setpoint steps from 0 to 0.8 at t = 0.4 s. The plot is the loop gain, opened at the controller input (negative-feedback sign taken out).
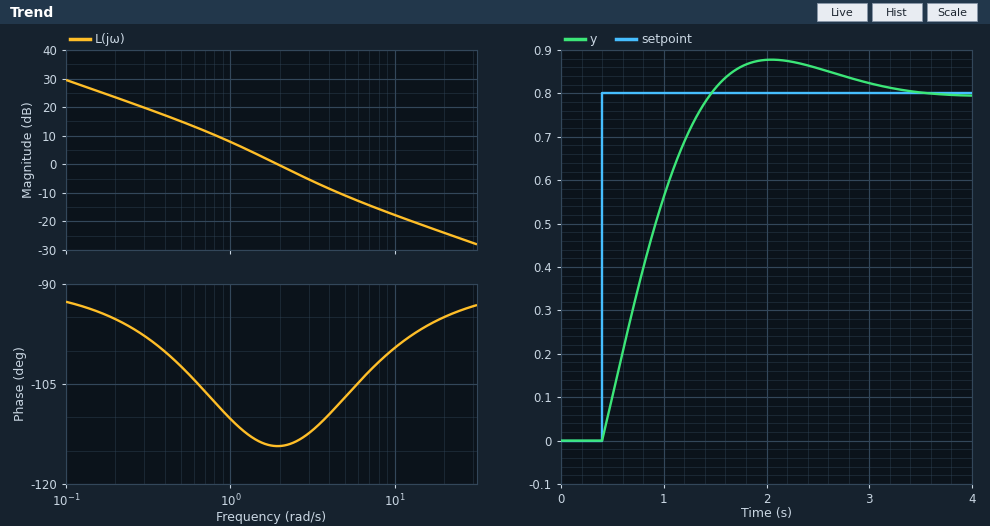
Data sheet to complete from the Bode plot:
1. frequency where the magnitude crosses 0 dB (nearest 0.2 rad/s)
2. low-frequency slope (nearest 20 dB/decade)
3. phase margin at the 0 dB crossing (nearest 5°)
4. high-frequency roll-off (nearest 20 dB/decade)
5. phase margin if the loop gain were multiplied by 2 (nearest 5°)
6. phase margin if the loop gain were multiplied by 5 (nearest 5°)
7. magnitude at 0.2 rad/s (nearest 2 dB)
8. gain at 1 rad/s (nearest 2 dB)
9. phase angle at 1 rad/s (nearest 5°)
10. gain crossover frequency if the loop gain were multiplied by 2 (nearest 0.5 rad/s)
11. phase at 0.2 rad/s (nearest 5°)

2.0 rad/s
-20 dB/decade
65°
-20 dB/decade
70°
75°
24 dB
8 dB
-110°
3.0 rad/s
-95°
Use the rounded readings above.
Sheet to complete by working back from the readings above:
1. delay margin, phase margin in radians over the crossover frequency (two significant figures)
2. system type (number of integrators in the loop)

0.57 s
1
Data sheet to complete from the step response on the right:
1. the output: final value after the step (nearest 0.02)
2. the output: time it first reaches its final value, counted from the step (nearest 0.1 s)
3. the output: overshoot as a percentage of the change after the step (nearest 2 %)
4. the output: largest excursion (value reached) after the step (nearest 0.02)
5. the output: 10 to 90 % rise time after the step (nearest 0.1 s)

0.80
1.1 s
10 %
0.88
0.8 s
